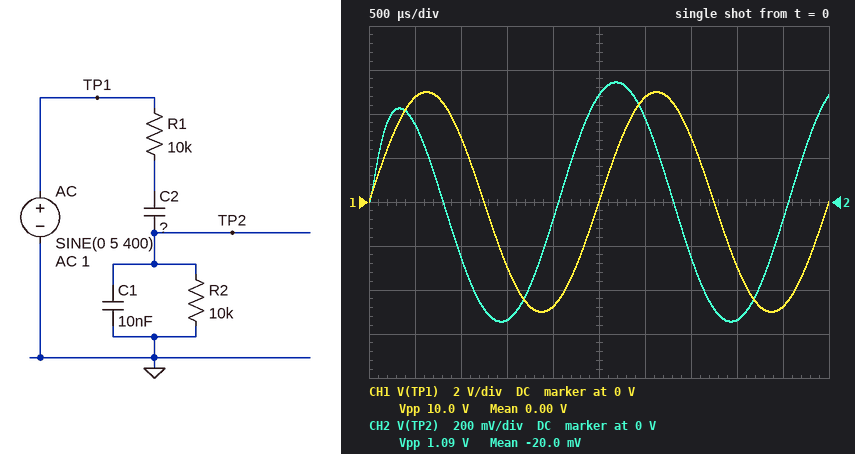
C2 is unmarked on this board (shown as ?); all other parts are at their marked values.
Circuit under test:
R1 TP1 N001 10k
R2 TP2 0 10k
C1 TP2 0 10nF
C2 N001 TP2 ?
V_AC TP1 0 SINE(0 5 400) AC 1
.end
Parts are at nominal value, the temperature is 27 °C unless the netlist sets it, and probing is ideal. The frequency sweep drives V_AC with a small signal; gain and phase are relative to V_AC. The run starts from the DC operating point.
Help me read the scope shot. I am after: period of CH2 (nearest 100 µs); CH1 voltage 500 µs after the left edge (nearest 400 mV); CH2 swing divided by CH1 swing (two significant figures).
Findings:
2.5 ms
4.8 V
0.11
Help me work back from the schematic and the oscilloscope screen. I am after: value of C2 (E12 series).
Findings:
4.7 nF
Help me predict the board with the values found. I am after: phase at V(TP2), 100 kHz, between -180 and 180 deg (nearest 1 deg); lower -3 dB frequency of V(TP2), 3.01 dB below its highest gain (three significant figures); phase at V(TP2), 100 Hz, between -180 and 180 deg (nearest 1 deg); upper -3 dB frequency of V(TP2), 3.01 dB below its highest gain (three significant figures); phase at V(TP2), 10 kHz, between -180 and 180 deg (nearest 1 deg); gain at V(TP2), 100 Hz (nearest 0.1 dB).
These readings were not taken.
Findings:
-86 deg
738 Hz
83 deg
7.31 kHz
-55 deg
-30.6 dB
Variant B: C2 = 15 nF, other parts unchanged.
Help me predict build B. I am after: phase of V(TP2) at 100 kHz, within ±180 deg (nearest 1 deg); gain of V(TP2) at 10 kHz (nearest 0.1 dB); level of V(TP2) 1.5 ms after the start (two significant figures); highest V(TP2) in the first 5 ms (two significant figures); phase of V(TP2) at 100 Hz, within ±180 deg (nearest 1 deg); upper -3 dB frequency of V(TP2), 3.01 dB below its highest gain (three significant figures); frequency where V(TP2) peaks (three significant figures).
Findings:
-88 deg
-16.6 dB
-1.4 V
1.4 V
76 deg
4.61 kHz
1.30 kHz
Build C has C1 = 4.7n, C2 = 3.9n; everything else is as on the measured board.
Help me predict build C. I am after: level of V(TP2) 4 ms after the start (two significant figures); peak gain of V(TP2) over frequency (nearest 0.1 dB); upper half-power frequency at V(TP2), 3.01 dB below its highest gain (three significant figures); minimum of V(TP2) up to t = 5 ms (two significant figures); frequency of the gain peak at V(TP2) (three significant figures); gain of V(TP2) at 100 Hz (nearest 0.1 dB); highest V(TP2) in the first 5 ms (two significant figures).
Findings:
-450 mV
-10.1 dB
12.0 kHz
-470 mV
3.72 kHz
-32.2 dB
470 mV
